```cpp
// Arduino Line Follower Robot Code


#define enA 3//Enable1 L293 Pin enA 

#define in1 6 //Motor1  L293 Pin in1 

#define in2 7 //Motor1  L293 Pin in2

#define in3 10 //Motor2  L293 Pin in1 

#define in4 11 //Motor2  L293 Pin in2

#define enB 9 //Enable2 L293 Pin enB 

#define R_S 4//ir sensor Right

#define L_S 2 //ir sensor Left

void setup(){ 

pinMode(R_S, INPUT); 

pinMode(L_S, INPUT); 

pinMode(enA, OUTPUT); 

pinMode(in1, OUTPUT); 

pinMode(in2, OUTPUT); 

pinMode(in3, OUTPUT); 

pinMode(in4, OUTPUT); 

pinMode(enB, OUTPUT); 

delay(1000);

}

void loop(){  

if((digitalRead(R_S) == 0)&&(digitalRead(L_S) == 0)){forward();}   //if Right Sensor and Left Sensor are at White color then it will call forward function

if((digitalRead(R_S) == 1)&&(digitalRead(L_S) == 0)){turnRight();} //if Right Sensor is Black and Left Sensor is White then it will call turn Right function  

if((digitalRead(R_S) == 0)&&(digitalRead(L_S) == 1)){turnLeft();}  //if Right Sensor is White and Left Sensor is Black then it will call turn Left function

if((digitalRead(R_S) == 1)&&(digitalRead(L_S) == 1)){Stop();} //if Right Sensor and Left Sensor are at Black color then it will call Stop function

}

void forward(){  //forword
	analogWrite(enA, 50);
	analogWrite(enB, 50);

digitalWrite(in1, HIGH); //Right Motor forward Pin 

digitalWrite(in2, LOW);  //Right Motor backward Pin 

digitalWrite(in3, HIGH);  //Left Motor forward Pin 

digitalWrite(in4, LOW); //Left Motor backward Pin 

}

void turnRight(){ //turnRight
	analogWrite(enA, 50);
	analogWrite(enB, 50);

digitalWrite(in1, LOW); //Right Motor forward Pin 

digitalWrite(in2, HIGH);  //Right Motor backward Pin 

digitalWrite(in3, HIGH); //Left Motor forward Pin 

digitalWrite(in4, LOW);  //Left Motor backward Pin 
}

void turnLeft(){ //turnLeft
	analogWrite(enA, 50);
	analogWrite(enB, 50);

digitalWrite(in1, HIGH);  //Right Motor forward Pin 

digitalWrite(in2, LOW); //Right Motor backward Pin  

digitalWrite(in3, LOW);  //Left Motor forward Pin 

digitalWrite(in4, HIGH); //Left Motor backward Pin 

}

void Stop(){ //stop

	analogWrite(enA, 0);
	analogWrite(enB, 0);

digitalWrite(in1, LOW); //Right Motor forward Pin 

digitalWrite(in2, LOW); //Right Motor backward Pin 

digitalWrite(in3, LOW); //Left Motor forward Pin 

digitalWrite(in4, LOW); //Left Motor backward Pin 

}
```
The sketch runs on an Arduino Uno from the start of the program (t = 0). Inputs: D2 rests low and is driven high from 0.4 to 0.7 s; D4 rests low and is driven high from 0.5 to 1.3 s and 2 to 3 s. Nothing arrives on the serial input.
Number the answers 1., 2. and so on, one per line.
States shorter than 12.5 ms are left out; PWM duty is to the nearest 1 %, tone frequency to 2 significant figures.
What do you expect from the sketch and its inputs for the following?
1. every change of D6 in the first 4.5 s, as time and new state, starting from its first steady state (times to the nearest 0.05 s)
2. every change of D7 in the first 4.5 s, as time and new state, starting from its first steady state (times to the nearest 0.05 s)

1. 0 s low; 1.3 s high; 2 s low; 3 s high
2. 0 s low; 1 s high; 1.3 s low; 2 s high; 3 s low
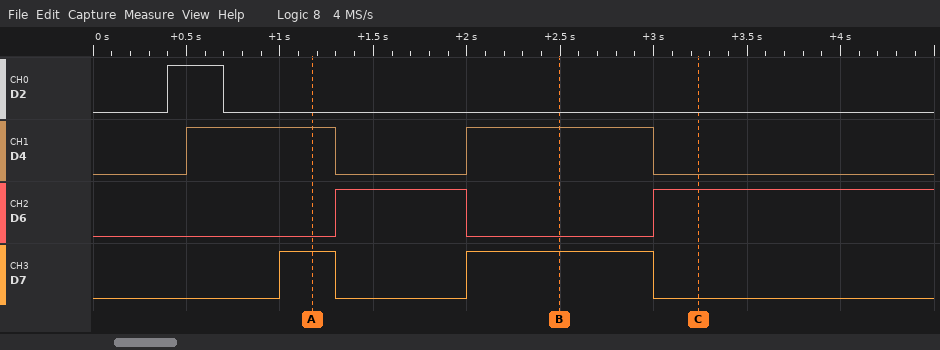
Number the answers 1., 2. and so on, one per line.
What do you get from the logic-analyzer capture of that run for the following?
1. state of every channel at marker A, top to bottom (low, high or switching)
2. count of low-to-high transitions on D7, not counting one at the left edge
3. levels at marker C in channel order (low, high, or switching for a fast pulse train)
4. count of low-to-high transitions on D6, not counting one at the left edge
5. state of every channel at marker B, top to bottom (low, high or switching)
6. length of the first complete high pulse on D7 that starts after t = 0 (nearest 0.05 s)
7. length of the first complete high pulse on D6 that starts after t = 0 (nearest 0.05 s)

1. D2 low, D4 high, D6 low, D7 high
2. 2
3. D2 low, D4 low, D6 high, D7 low
4. 2
5. D2 low, D4 high, D6 low, D7 high
6. 0.30 s
7. 0.70 s
